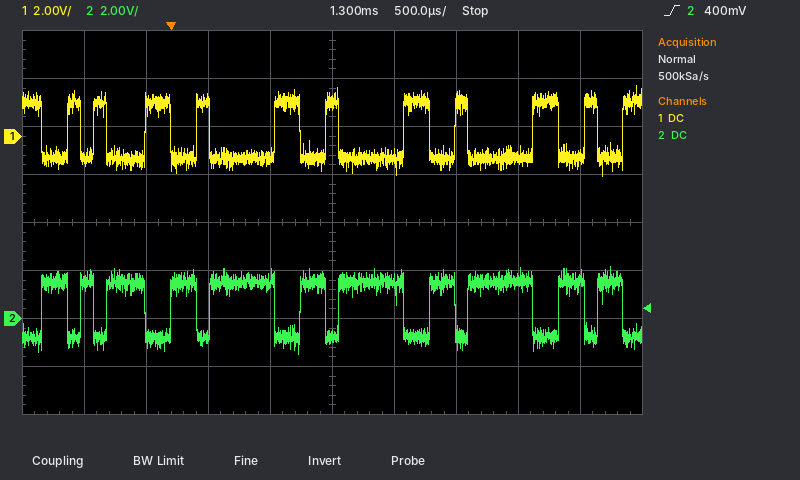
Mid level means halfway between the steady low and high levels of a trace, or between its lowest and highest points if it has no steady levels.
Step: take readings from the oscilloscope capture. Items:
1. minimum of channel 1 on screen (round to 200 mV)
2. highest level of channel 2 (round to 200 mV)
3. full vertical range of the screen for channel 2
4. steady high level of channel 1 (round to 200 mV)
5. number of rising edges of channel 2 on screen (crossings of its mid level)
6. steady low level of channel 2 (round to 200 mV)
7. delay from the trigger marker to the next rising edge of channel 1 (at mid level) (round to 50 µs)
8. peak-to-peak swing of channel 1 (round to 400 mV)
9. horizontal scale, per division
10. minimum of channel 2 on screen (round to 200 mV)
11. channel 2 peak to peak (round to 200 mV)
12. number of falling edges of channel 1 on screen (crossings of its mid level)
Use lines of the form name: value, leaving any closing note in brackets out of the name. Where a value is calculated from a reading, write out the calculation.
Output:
minimum of channel 1 on screen: -1.6 V
highest level of channel 2: 2.2 V
full vertical range of the screen for channel 2: 16 V
steady high level of channel 1: 1.4 V
number of rising edges of channel 2 on screen: 11
steady low level of channel 2: -800 mV
delay from the trigger marker to the next rising edge of channel 1 (at mid level): 200 µs
peak-to-peak swing of channel 1: 3.6 V
horizontal scale, per division: 500 µs
minimum of channel 2 on screen: -1.4 V
channel 2 peak to peak: 2.2 V − (-1.4 V) = 3.6 V
number of falling edges of channel 1 on screen: 11
